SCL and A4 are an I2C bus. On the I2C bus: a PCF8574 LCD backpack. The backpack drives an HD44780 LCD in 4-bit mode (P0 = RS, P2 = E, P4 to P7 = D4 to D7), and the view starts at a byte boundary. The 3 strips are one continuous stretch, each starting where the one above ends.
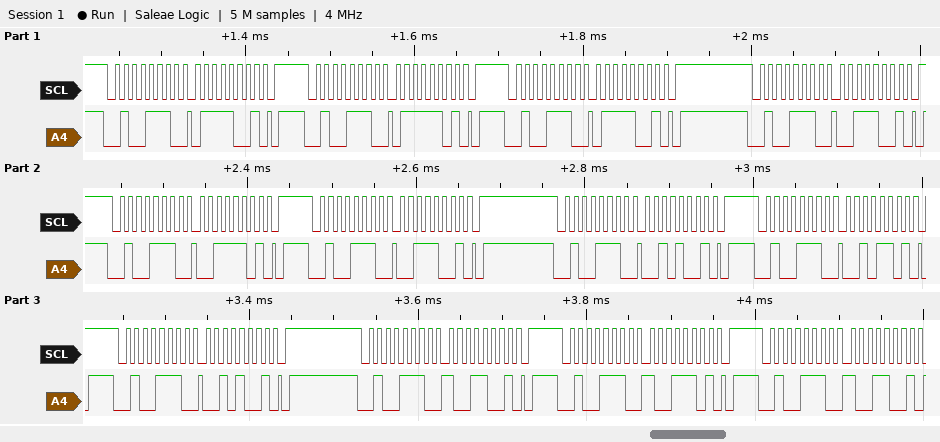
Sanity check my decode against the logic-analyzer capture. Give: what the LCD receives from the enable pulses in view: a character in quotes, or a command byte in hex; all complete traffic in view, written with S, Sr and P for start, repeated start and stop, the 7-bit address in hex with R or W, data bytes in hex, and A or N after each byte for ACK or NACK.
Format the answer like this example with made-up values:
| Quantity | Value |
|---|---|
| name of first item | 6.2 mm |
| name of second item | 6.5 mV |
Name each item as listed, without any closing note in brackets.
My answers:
| Quantity | Value |
|---|---|
| what the LCD receives from the enable pulses in view: a character in quotes, or a command byte in hex | 's' ')' |
| all complete traffic in view, written with S, Sr and P for start, repeated start and stop, the 7-bit address in hex with R or W, data bytes in hex, and A or N after each byte for ACK or NACK | S 27W A 79 A P S 27W A 7D A P S 27W A 79 A P S 27W A 39 A P S 27W A 3D A P S 27W A 39 A P S 27W A 29 A P S 27W A 2D A P S 27W A 29 A P S 27W A 99 A P S 27W A 9D A P S 27W A 99 A |
